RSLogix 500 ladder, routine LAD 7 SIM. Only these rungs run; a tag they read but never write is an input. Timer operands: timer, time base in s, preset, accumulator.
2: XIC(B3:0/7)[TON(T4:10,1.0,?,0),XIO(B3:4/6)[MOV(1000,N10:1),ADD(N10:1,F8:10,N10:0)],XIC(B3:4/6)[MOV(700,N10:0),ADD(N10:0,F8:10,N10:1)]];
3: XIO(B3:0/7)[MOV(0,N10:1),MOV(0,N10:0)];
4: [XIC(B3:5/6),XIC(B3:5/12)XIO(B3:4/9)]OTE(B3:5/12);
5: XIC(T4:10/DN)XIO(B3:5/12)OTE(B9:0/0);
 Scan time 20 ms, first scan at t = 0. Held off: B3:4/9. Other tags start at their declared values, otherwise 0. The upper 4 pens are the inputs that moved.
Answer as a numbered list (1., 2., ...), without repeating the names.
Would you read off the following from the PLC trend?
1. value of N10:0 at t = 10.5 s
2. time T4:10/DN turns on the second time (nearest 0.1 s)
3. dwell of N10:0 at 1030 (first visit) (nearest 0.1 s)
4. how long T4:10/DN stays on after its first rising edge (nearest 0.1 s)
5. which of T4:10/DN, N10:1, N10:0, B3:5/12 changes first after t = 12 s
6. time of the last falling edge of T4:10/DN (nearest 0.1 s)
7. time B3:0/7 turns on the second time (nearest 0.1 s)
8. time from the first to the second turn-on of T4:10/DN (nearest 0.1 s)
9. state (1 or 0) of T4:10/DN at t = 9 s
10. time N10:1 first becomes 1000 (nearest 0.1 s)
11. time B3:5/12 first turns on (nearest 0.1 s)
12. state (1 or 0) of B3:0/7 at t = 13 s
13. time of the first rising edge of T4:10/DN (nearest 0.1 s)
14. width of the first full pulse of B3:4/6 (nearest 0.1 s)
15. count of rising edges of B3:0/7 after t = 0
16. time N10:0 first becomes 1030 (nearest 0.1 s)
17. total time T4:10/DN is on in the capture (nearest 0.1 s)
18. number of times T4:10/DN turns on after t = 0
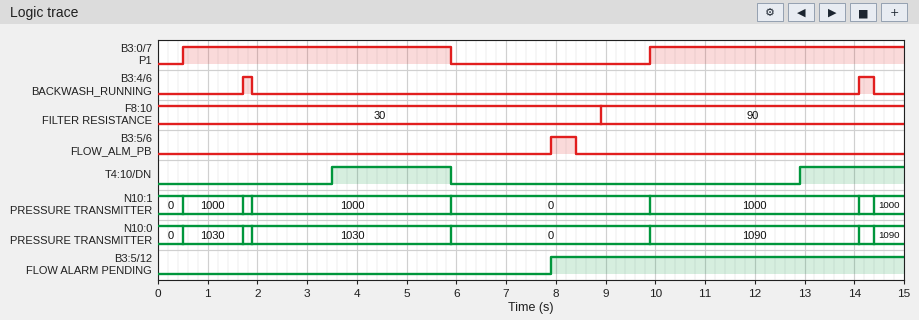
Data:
1. 1090
2. 12.9 s
3. 1.2 s
4. 2.4 s
5. T4:10/DN
6. 5.9 s
7. 9.9 s
8. 9.4 s
9. 0
10. 0.5 s
11. 7.9 s
12. 1
13. 3.5 s
14. 0.2 s
15. 2
16. 0.5 s
17. 4.5 s
18. 2
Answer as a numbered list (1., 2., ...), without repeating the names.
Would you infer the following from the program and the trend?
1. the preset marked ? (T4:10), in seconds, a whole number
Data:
1. 3 s
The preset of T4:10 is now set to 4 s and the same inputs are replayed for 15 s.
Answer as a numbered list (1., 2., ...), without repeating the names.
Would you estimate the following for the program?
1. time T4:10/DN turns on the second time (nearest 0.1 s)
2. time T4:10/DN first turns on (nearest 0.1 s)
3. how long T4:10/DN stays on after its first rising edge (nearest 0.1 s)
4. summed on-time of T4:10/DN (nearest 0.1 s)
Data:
1. 13.9 s
2. 4.5 s
3. 1.4 s
4. 2.5 s
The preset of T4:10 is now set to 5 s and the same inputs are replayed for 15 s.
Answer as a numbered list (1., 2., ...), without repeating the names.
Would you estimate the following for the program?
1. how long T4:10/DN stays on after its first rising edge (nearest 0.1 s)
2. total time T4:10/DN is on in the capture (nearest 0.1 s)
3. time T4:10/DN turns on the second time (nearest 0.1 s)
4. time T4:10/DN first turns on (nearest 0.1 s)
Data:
1. 0.4 s
2. 0.5 s
3. 14.9 s
4. 5.5 s
